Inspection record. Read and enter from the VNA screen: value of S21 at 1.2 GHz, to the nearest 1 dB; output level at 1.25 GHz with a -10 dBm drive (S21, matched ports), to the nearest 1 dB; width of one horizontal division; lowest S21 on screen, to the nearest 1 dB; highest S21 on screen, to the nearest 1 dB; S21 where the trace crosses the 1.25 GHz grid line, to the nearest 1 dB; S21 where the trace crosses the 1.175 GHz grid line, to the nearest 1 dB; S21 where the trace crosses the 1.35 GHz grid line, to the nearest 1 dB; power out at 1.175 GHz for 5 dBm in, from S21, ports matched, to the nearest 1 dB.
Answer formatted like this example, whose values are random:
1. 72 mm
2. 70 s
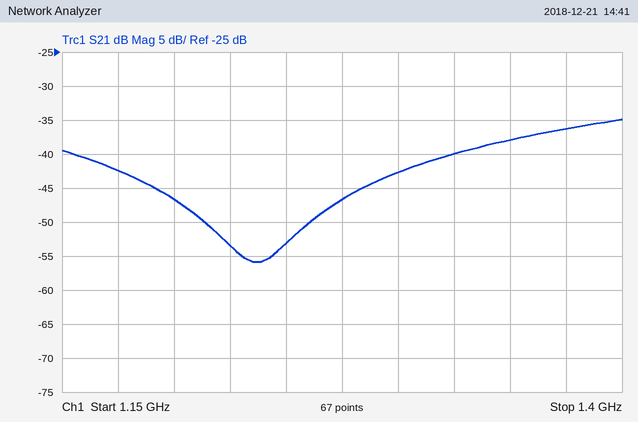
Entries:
1. -47 dB
2. -63 dBm
3. 25 MHz
4. -56 dB
5. -35 dB
6. -53 dB
7. -42 dB
8. -38 dB
9. -37 dBm
